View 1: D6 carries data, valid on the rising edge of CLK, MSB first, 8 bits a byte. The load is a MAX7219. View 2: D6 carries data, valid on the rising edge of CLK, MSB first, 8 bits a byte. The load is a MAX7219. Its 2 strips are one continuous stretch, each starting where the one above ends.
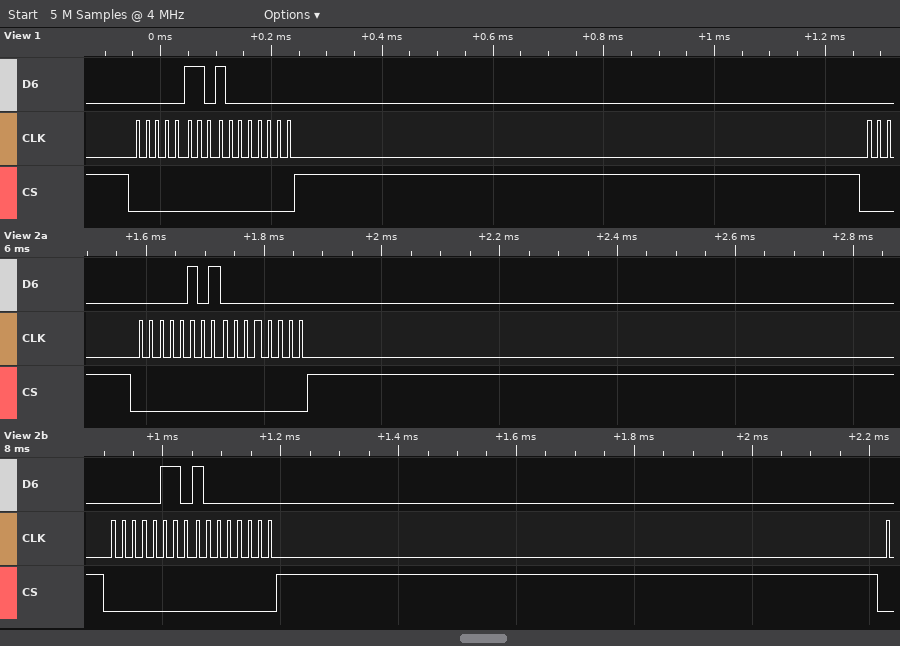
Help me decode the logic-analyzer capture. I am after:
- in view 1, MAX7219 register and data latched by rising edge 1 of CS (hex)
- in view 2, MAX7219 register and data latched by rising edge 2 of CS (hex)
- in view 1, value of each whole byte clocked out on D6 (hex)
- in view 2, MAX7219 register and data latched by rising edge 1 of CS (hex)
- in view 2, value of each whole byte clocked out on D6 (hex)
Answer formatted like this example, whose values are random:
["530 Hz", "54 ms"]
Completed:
["register 0x6, data 0x80", "register 0x6, data 0x80", "06 80", "register 0x5, data 0x00", "0x05 0x00 0x06 0x80"]
